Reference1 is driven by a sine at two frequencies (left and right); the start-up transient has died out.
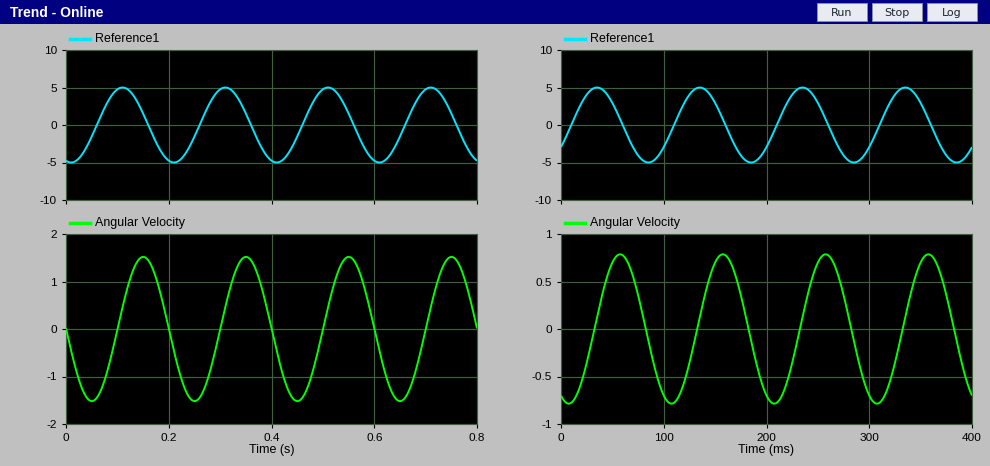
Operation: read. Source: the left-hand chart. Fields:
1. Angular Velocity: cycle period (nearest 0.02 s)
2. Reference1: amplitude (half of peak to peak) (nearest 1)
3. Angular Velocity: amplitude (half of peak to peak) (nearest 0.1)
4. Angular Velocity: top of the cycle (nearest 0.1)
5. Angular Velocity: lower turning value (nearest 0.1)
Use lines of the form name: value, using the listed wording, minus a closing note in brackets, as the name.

Angular Velocity: cycle period: 0.20 s
Reference1: amplitude (half of peak to peak): 5
Angular Velocity: amplitude (half of peak to peak): 1.5
Angular Velocity: top of the cycle: 1.5
Angular Velocity: lower turning value: -1.5
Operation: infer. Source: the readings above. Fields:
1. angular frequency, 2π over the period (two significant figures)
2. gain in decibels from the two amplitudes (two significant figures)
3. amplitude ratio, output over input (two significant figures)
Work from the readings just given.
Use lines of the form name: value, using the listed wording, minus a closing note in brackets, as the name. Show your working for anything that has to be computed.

angular frequency, 2π over the period: 2π / 0.2 = 31 rad/s
gain in decibels from the two amplitudes: 20 log10(1.5 / 5) = -10 dB
amplitude ratio, output over input: 1.5 / 5 = 0.30
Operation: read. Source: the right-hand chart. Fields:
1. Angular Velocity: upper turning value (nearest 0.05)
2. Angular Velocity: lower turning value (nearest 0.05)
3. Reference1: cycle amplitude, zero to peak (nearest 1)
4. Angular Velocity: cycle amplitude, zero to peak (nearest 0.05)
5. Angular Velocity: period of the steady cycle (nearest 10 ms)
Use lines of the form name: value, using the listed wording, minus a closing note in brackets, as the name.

Angular Velocity: upper turning value: 0.80
Angular Velocity: lower turning value: -0.80
Reference1: cycle amplitude, zero to peak: 5
Angular Velocity: cycle amplitude, zero to peak: 0.80
Angular Velocity: period of the steady cycle: 100 ms
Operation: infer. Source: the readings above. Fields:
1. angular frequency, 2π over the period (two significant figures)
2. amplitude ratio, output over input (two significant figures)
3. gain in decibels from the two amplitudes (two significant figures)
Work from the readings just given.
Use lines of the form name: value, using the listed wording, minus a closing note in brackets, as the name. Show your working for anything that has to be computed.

angular frequency, 2π over the period: 2π / 100 = 0.063 rad/ms
amplitude ratio, output over input: 0.8 / 5 = 0.16
gain in decibels from the two amplitudes: 20 log10(0.8 / 5) = -16 dB
